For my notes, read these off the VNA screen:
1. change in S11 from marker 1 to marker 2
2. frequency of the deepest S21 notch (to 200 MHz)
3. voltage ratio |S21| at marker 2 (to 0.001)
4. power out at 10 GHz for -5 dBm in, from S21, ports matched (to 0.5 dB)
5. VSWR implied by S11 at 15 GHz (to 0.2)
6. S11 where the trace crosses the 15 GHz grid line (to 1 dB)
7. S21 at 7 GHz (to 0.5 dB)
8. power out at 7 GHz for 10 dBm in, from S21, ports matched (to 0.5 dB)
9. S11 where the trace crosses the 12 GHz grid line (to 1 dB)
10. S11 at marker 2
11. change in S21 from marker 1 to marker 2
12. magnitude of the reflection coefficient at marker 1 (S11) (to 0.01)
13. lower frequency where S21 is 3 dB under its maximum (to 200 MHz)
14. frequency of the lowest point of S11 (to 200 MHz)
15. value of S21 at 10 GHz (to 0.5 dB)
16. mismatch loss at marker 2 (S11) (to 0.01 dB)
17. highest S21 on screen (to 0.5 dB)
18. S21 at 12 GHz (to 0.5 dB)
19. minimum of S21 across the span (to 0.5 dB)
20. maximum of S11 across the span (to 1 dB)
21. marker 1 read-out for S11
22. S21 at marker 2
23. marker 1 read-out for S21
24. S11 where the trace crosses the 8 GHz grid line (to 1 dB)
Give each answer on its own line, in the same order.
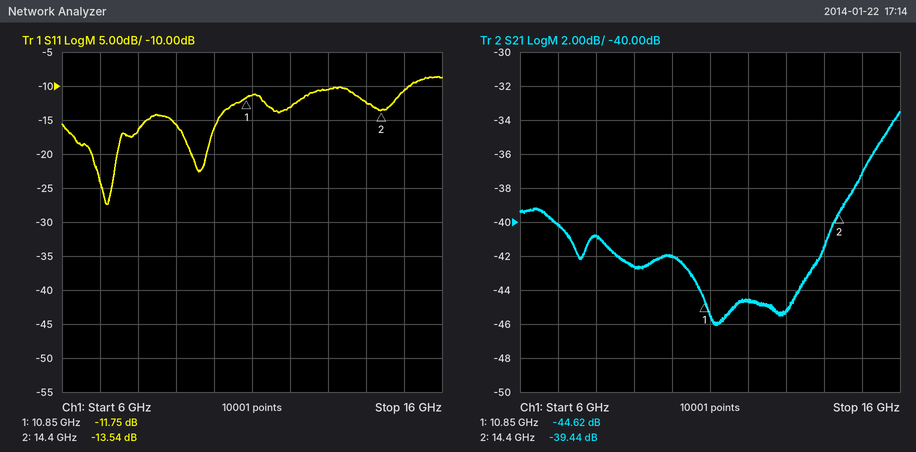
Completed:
-1.79 dB
11.2 GHz
0.011
-47.0 dBm
1.8
-11 dB
-40.0 dB
-30.0 dBm
-13 dB
-13.54 dB
5.18 dB
0.26
15.2 GHz
7.2 GHz
-42.0 dB
0.20 dB
-33.5 dB
-44.5 dB
-46.0 dB
-9 dB
-11.75 dB
-39.44 dB
-44.62 dB
-17 dB
